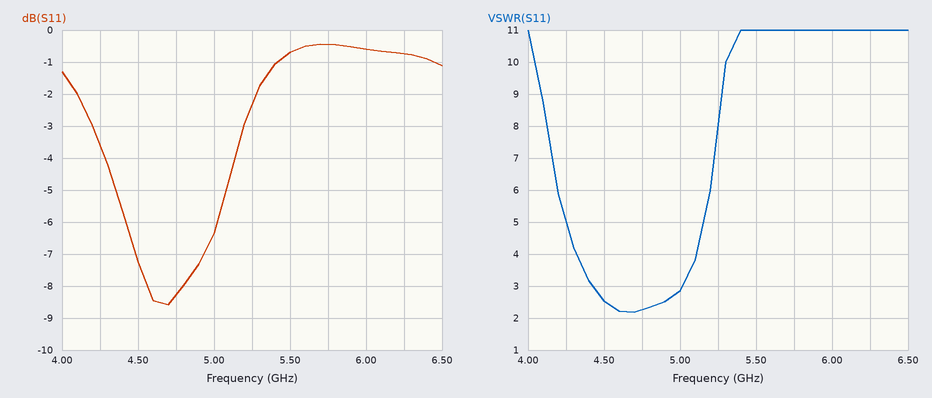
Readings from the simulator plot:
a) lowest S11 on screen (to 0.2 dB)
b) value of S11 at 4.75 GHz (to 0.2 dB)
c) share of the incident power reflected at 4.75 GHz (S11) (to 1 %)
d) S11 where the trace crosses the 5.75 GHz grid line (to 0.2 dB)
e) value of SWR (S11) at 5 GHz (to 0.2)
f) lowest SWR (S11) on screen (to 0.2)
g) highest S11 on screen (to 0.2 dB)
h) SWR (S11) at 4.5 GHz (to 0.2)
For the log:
-8.6 dB
-8.2 dB
15 %
-0.4 dB
2.8
2.2
-0.4 dB
2.6
